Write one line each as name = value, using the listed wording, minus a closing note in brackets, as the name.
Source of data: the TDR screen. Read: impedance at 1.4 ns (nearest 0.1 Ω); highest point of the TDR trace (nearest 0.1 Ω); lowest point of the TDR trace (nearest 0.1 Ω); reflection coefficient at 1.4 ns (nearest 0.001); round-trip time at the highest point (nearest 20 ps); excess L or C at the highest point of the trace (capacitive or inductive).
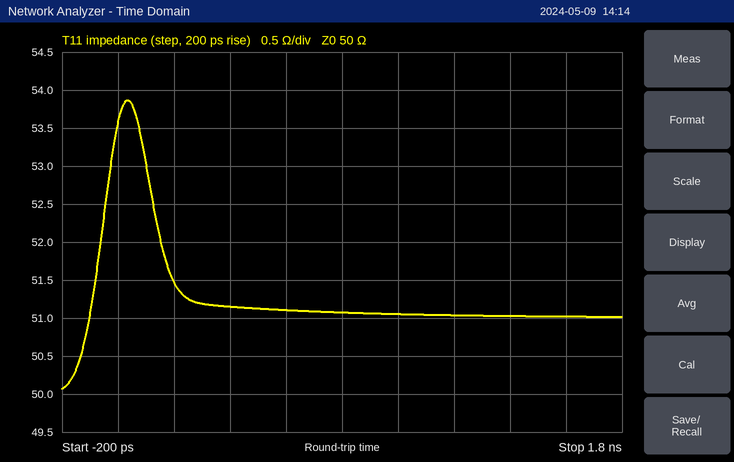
impedance at 1.4 ns = 51.0 Ω
highest point of the TDR trace = 53.9 Ω
lowest point of the TDR trace = 50.1 Ω
reflection coefficient at 1.4 ns = +0.010
round-trip time at the highest point = 40 ps
excess L or C at the highest point of the trace = inductive
